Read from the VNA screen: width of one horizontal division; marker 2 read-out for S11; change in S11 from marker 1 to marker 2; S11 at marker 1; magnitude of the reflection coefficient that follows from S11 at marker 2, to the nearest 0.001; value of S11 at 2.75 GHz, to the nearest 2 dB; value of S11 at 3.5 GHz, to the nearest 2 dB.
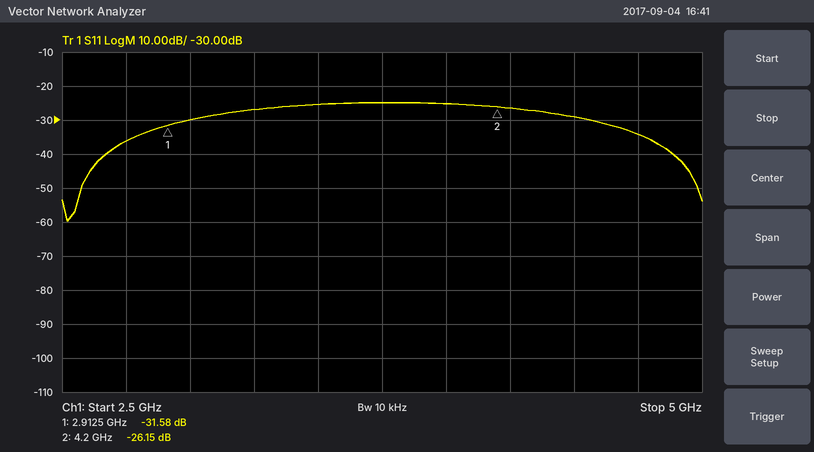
250 MHz
-26.15 dB
5.43 dB
-31.58 dB
0.049
-36 dB
-26 dB
